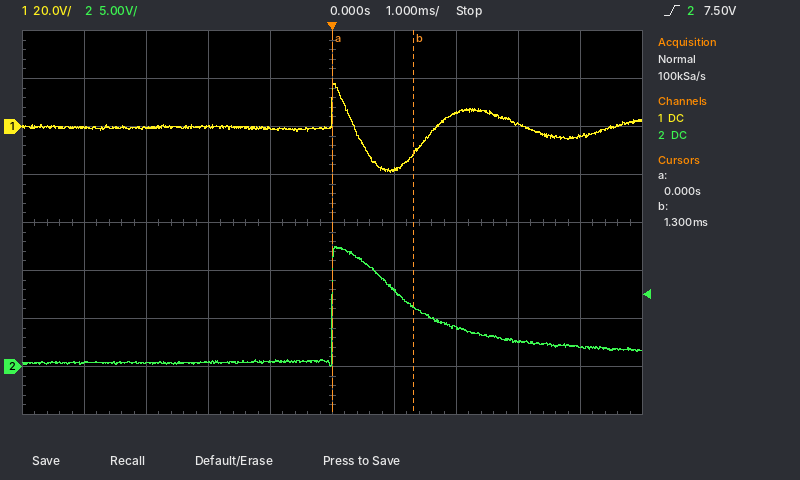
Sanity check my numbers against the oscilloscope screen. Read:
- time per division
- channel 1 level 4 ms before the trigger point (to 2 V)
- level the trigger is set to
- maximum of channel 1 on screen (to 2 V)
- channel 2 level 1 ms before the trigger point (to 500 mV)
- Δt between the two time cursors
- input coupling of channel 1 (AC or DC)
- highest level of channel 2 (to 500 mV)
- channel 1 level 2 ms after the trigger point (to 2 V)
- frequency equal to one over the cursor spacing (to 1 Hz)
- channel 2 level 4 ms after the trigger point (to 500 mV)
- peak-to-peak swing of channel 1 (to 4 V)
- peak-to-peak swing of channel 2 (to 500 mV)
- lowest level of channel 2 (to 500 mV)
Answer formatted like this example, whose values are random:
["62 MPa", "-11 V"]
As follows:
["1 ms", "0 V", "7.50 V", "18 V", "500 mV", "1.3 ms", "DC", "12.5 V", "6 V", "769 Hz", "2.0 V", "36 V", "12.5 V", "0.0 V"]
